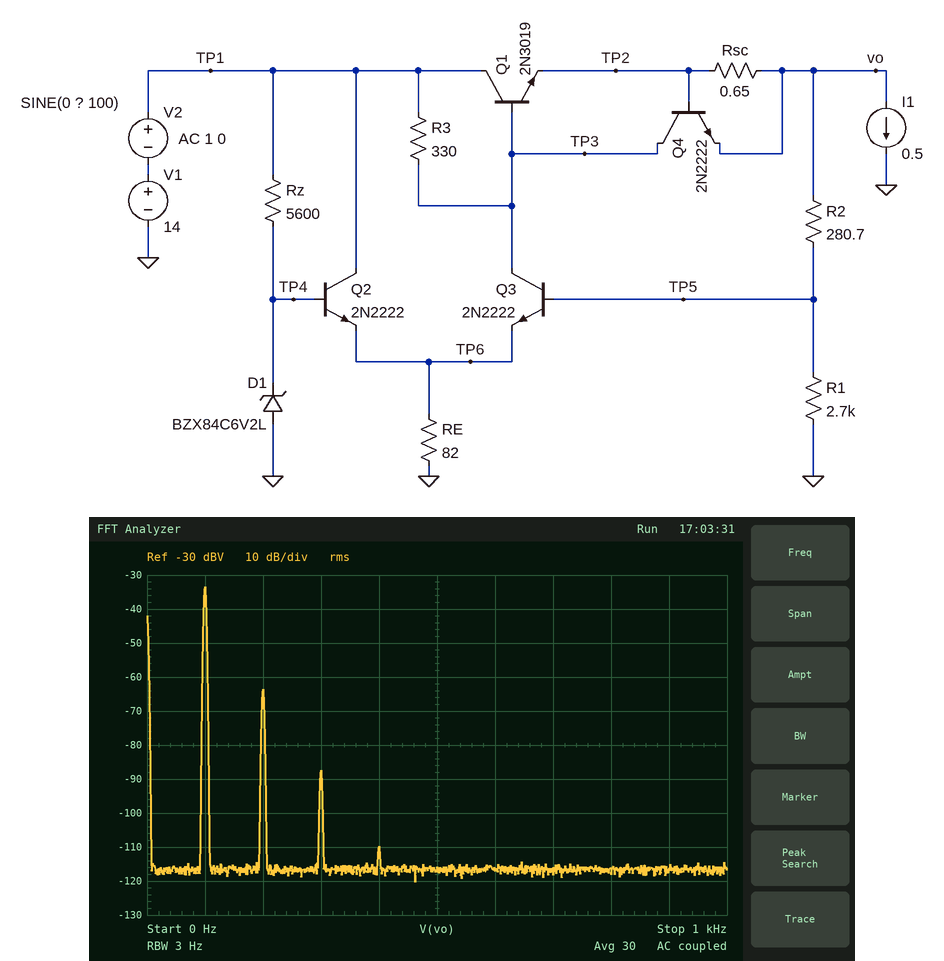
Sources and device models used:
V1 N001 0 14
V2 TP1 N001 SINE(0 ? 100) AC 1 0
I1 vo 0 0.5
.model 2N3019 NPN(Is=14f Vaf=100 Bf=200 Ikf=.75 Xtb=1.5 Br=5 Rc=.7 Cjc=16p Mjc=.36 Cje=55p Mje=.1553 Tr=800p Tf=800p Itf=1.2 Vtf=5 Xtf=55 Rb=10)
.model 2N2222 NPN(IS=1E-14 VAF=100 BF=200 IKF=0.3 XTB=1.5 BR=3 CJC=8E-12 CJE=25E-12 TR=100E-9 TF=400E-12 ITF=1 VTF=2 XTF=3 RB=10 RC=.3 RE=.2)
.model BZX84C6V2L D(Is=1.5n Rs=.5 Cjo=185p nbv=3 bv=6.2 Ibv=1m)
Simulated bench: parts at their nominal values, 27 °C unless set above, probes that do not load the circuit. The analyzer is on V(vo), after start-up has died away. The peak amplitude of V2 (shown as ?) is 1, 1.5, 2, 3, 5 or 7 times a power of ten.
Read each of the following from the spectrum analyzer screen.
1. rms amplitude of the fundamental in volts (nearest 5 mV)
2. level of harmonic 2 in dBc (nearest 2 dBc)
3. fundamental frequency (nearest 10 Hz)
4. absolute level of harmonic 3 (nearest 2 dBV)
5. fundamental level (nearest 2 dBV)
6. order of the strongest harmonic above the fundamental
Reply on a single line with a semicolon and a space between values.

20 mV; -30 dBc; 100 Hz; -88 dBV; -34 dBV; 2
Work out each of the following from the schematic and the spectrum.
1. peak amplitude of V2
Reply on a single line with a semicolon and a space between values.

1 V
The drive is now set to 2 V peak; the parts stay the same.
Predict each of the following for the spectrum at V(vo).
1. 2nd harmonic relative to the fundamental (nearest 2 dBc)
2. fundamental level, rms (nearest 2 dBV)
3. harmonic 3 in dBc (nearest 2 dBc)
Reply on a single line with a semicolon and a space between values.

-24 dBc; -28 dBV; -42 dBc
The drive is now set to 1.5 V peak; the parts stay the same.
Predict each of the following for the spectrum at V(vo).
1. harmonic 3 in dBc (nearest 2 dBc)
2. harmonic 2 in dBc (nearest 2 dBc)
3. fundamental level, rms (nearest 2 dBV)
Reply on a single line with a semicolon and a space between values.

-46 dBc; -26 dBc; -30 dBV
